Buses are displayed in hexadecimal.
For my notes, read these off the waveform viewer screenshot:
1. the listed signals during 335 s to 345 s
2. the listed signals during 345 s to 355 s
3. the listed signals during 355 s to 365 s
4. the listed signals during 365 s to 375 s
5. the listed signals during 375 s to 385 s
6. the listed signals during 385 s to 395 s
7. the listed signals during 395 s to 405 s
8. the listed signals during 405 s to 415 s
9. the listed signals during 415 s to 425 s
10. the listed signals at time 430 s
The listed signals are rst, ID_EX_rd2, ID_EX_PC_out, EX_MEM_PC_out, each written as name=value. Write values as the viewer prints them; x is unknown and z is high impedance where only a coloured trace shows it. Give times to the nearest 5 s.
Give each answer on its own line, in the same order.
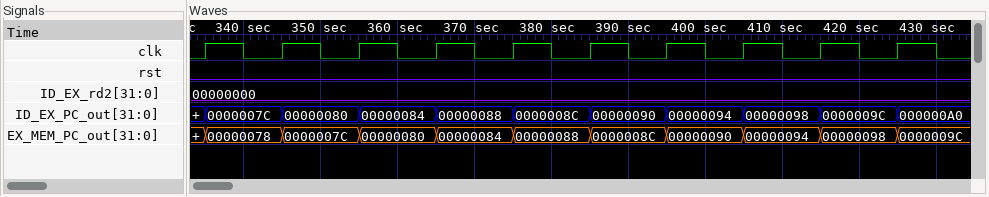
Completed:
rst=0, ID_EX_rd2=00000000, ID_EX_PC_out=0000007C, EX_MEM_PC_out=00000078
rst=0, ID_EX_rd2=00000000, ID_EX_PC_out=00000080, EX_MEM_PC_out=0000007C
rst=0, ID_EX_rd2=00000000, ID_EX_PC_out=00000084, EX_MEM_PC_out=00000080
rst=0, ID_EX_rd2=00000000, ID_EX_PC_out=00000088, EX_MEM_PC_out=00000084
rst=0, ID_EX_rd2=00000000, ID_EX_PC_out=0000008C, EX_MEM_PC_out=00000088
rst=0, ID_EX_rd2=00000000, ID_EX_PC_out=00000090, EX_MEM_PC_out=0000008C
rst=0, ID_EX_rd2=00000000, ID_EX_PC_out=00000094, EX_MEM_PC_out=00000090
rst=0, ID_EX_rd2=00000000, ID_EX_PC_out=00000098, EX_MEM_PC_out=00000094
rst=0, ID_EX_rd2=00000000, ID_EX_PC_out=0000009C, EX_MEM_PC_out=00000098
rst=0, ID_EX_rd2=00000000, ID_EX_PC_out=000000A0, EX_MEM_PC_out=0000009C
